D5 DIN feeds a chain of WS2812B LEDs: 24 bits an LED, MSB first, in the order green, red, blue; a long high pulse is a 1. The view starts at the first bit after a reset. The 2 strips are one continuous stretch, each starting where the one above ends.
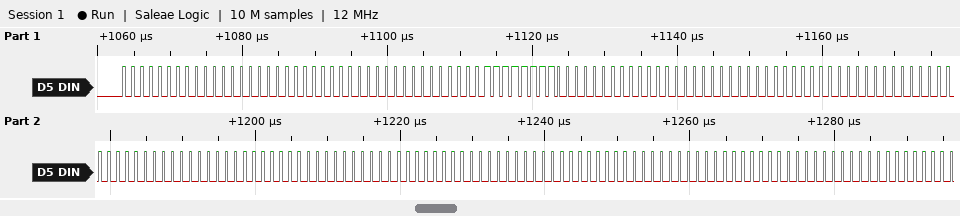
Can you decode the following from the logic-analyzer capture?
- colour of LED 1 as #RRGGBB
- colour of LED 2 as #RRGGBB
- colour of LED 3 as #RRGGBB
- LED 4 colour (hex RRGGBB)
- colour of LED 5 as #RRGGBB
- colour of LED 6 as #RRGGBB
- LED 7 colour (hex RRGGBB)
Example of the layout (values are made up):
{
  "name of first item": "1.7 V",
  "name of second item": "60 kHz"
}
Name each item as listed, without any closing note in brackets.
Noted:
{
  "colour of LED 1 as #RRGGBB": "#000000",
  "colour of LED 2 as #RRGGBB": "#0000FF",
  "colour of LED 3 as #RRGGBB": "#000000",
  "LED 4 colour": "#000000",
  "colour of LED 5 as #RRGGBB": "#000000",
  "colour of LED 6 as #RRGGBB": "#000000",
  "LED 7 colour": "#000000"
}
